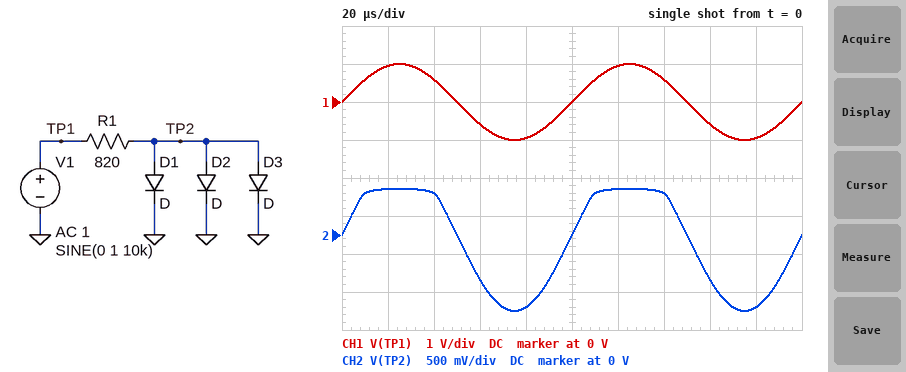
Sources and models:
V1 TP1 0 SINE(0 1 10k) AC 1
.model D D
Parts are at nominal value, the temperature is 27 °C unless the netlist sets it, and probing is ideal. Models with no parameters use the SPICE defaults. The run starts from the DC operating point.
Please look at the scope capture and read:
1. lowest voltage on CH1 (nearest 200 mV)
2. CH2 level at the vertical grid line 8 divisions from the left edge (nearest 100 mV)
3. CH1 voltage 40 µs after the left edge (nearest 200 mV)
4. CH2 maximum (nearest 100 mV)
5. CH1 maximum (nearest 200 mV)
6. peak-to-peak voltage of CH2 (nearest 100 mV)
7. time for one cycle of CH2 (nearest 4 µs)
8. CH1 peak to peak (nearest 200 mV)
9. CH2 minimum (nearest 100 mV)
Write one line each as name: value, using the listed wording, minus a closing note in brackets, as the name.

lowest voltage on CH1: -1.0 V
CH2 level at the vertical grid line 8 divisions from the left edge: -600 mV
CH1 voltage 40 µs after the left edge: 600 mV
CH2 maximum: 600 mV
CH1 maximum: 1.0 V
peak-to-peak voltage of CH2: 1.6 V
time for one cycle of CH2: 100 µs
CH1 peak to peak: 2.0 V
CH2 minimum: -1.0 V
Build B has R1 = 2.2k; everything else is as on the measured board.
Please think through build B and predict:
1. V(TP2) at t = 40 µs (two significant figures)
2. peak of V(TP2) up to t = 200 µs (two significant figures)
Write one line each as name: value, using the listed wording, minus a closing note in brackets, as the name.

V(TP2) at t = 40 µs: 530 mV
peak of V(TP2) up to t = 200 µs: 580 mV
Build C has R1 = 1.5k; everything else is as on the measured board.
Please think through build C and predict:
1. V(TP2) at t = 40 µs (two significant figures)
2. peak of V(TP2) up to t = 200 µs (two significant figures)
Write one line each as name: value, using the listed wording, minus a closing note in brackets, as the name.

V(TP2) at t = 40 µs: 540 mV
peak of V(TP2) up to t = 200 µs: 590 mV
